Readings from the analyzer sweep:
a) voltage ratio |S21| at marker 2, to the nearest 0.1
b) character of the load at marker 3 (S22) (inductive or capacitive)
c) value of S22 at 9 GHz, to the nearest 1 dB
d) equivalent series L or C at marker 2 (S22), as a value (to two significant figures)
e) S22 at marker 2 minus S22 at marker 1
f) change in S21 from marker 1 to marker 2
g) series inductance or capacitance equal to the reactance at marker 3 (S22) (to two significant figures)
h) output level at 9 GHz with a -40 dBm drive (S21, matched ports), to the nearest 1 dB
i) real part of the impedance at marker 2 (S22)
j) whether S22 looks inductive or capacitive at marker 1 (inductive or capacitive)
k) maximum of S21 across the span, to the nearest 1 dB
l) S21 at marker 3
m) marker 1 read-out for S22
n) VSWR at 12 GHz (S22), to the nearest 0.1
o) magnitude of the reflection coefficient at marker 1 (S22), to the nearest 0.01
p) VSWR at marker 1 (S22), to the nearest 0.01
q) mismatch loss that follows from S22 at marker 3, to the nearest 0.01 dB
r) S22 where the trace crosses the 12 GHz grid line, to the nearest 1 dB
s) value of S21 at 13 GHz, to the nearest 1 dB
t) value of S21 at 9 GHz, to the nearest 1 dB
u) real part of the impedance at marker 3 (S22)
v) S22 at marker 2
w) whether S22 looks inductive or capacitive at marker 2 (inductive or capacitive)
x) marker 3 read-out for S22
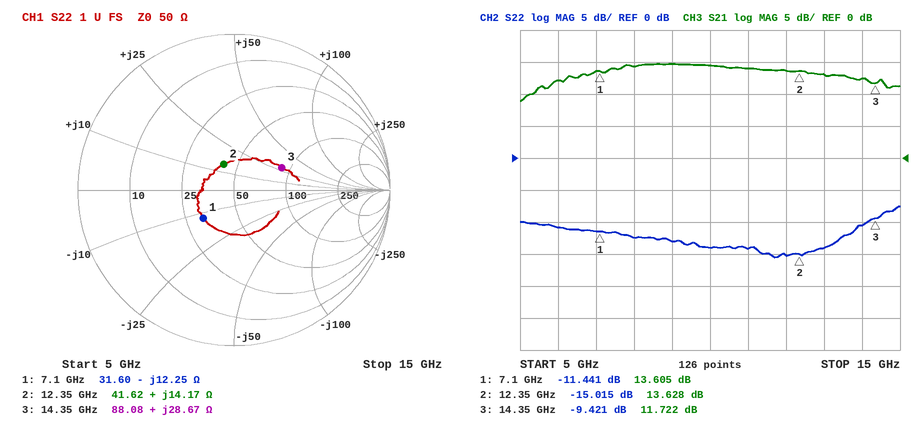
4.8
inductive
-13 dB
180 pH
-3.574 dB
0.023 dB
320 pH
-25 dBm
41.62 Ω
capacitive
15 dB
11.722 dB
-11.441 dB
1.4
0.27
1.73
0.53 dB
-15 dB
13 dB
15 dB
88.08 Ω
-15.015 dB
inductive
-9.421 dB
